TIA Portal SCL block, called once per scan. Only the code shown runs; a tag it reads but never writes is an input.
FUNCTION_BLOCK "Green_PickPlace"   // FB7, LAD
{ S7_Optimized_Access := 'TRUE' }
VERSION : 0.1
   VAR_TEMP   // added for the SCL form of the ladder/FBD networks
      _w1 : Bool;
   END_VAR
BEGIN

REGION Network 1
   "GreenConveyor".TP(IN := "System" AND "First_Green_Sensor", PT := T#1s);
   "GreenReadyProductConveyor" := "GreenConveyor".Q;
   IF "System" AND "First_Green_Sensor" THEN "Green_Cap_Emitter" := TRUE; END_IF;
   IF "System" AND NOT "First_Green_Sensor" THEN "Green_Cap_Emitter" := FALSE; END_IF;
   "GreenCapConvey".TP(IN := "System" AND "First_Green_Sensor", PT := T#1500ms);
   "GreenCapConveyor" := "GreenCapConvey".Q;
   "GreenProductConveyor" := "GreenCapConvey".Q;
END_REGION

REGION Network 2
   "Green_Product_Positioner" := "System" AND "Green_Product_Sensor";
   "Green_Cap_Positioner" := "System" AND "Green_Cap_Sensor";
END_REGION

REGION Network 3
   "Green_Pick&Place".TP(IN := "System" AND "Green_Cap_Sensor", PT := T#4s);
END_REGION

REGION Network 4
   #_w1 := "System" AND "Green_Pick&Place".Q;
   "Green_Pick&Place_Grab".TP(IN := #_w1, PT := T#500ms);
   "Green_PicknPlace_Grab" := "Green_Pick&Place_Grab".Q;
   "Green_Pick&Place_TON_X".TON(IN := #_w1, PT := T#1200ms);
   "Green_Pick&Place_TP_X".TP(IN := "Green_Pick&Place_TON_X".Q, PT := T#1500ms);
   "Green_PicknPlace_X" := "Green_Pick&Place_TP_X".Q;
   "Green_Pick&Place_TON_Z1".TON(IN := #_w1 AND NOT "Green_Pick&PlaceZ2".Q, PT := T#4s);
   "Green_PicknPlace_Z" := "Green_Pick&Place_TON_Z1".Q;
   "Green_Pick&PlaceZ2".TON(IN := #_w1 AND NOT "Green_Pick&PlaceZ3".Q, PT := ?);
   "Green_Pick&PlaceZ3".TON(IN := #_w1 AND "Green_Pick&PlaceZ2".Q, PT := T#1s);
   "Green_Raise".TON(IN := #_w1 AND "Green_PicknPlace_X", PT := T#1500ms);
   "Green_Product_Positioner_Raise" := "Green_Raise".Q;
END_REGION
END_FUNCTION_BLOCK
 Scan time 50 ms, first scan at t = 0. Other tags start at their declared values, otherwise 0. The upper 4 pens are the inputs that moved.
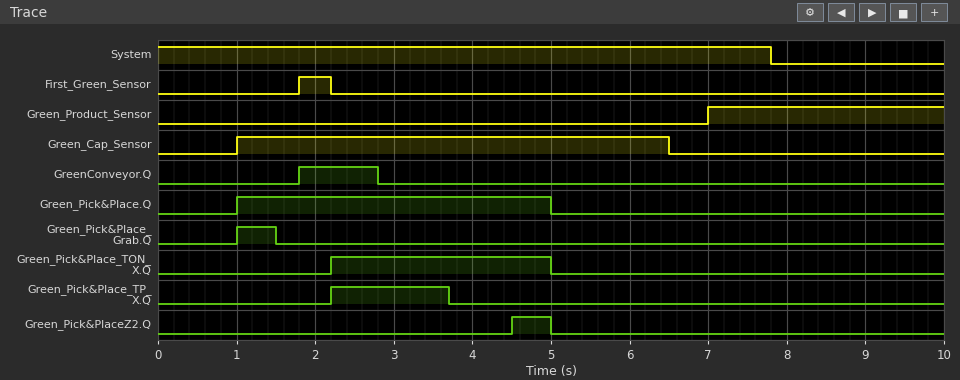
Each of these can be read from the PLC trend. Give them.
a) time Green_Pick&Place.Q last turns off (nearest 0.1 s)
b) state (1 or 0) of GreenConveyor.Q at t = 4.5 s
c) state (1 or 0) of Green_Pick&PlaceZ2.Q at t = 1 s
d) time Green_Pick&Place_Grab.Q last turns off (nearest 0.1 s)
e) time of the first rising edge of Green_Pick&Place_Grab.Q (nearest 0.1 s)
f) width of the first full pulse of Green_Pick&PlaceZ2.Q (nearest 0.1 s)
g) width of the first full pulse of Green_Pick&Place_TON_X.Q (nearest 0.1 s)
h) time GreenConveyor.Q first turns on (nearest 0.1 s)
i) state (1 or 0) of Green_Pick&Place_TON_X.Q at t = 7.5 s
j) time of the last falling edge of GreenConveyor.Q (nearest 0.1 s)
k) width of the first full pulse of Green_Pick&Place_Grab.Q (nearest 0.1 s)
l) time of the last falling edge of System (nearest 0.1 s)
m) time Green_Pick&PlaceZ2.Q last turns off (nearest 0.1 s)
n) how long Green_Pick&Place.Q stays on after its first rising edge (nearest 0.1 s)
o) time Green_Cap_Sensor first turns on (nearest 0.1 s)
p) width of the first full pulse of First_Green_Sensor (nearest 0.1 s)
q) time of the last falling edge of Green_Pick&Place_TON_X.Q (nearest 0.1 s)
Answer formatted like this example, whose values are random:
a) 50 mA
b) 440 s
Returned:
a) 5.0 s
b) 0
c) 0
d) 1.5 s
e) 1.0 s
f) 0.5 s
g) 2.8 s
h) 1.8 s
i) 0
j) 2.8 s
k) 0.5 s
l) 7.8 s
m) 5.0 s
n) 4.0 s
o) 1.0 s
p) 0.4 s
q) 5.0 s
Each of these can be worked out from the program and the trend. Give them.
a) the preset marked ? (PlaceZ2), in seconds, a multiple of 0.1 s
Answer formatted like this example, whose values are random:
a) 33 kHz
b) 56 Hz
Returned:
a) 3.5 s
